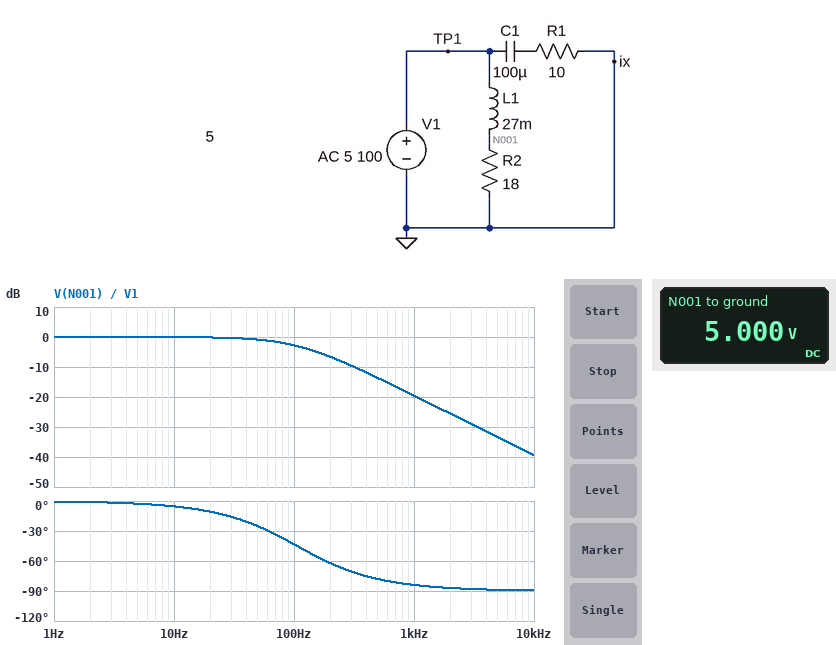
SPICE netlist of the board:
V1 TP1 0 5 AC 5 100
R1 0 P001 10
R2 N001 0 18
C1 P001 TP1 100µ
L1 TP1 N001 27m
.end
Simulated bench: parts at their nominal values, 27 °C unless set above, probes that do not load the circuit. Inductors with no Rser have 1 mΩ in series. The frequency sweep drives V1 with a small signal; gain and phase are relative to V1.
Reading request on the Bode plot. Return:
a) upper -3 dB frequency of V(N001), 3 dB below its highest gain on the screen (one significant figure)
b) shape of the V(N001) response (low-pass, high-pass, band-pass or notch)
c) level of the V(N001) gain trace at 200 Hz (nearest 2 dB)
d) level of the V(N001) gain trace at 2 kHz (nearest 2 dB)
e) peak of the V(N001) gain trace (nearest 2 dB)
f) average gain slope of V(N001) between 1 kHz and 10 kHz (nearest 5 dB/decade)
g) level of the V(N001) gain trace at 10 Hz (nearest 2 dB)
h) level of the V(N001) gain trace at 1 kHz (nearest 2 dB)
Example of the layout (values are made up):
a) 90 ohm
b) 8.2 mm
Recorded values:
a) 100 Hz
b) low-pass
c) -6 dB
d) -26 dB
e) 0 dB
f) -20 dB/decade
g) 0 dB
h) -20 dB
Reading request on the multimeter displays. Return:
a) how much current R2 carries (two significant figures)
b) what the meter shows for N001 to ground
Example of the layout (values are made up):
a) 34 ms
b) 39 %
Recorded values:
a) 280 mA
b) 5.000 V
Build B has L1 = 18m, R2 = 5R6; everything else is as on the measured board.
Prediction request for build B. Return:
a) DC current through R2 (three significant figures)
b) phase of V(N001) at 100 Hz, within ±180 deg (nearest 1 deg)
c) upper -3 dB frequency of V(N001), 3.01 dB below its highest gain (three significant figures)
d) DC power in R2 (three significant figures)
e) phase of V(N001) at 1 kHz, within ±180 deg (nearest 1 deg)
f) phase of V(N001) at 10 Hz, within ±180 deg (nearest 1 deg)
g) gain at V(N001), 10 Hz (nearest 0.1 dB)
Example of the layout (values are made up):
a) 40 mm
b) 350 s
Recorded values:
a) 893 mA
b) -64 deg
c) 49.5 Hz
d) 4.46 W
e) -87 deg
f) -11 deg
g) -0.2 dB
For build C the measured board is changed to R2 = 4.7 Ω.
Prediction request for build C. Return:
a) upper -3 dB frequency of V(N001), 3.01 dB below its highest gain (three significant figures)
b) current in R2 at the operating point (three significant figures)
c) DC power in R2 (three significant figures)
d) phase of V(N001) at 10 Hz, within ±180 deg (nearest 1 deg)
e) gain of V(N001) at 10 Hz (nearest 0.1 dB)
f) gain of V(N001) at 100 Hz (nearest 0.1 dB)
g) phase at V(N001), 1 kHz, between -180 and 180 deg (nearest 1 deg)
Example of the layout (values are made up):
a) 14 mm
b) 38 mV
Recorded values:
a) 27.7 Hz
b) 1.06 A
c) 5.32 W
d) -20 deg
e) -0.5 dB
f) -11.5 dB
g) -88 deg
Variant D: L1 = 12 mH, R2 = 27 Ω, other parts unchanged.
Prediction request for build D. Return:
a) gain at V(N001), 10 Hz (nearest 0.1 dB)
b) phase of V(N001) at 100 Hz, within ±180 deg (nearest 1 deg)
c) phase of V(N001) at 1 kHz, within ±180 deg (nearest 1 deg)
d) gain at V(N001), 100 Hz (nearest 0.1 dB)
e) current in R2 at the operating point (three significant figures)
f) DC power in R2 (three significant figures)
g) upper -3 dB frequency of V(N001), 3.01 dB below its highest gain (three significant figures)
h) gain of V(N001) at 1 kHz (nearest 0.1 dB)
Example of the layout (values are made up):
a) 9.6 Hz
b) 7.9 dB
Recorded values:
a) 0 dB
b) -16 deg
c) -70 deg
d) -0.3 dB
e) 185 mA
f) 926 mW
g) 358 Hz
h) -9.4 dB
